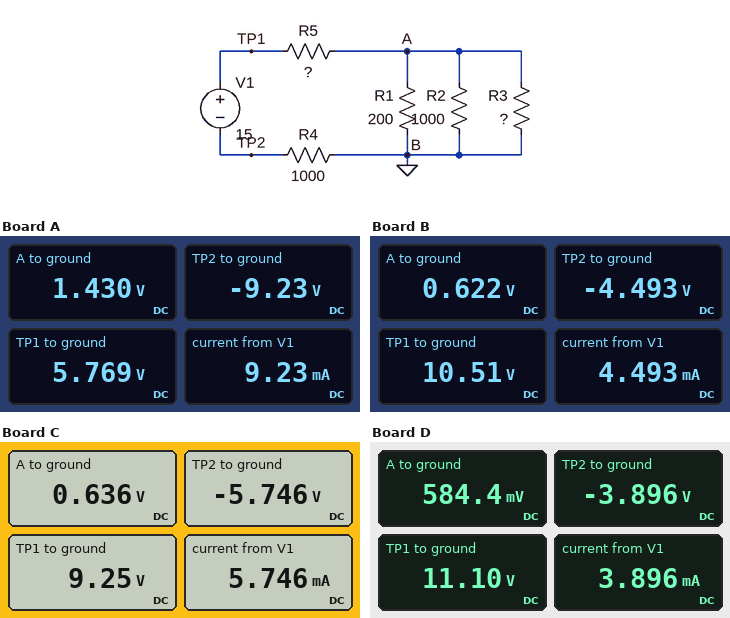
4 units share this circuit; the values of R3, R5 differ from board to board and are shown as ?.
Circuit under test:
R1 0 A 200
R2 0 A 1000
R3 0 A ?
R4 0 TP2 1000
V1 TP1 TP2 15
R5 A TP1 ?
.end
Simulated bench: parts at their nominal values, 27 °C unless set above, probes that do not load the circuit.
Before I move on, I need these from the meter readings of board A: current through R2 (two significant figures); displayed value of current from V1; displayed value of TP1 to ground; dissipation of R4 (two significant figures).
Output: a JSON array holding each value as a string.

["1.4 mA", "9.23 mA", "5.769 V", "85 mW"]
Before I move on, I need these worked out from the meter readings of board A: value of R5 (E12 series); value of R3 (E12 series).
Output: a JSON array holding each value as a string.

["470 Ω", "2.2 kΩ"]
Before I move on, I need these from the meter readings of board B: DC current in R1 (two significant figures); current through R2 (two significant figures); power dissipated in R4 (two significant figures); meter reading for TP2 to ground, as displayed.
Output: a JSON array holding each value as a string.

["3.1 mA", "620 µA", "20 mW", "-4.493 V"]
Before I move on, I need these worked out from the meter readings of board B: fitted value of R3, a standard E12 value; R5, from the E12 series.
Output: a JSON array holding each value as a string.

["820 Ω", "2.2 kΩ"]
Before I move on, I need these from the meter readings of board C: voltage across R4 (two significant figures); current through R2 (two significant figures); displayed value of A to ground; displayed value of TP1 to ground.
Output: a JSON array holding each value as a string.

["5.7 V", "640 µA", "0.636 V", "9.25 V"]
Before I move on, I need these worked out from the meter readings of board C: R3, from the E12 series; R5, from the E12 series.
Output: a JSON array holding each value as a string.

["330 Ω", "1.5 kΩ"]
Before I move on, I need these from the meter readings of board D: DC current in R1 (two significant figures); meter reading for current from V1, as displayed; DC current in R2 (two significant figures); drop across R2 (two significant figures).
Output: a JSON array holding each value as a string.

["2.9 mA", "3.896 mA", "580 µA", "580 mV"]
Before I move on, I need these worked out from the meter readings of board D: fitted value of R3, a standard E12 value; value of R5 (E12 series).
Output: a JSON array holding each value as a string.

["1.5 kΩ", "2.7 kΩ"]
